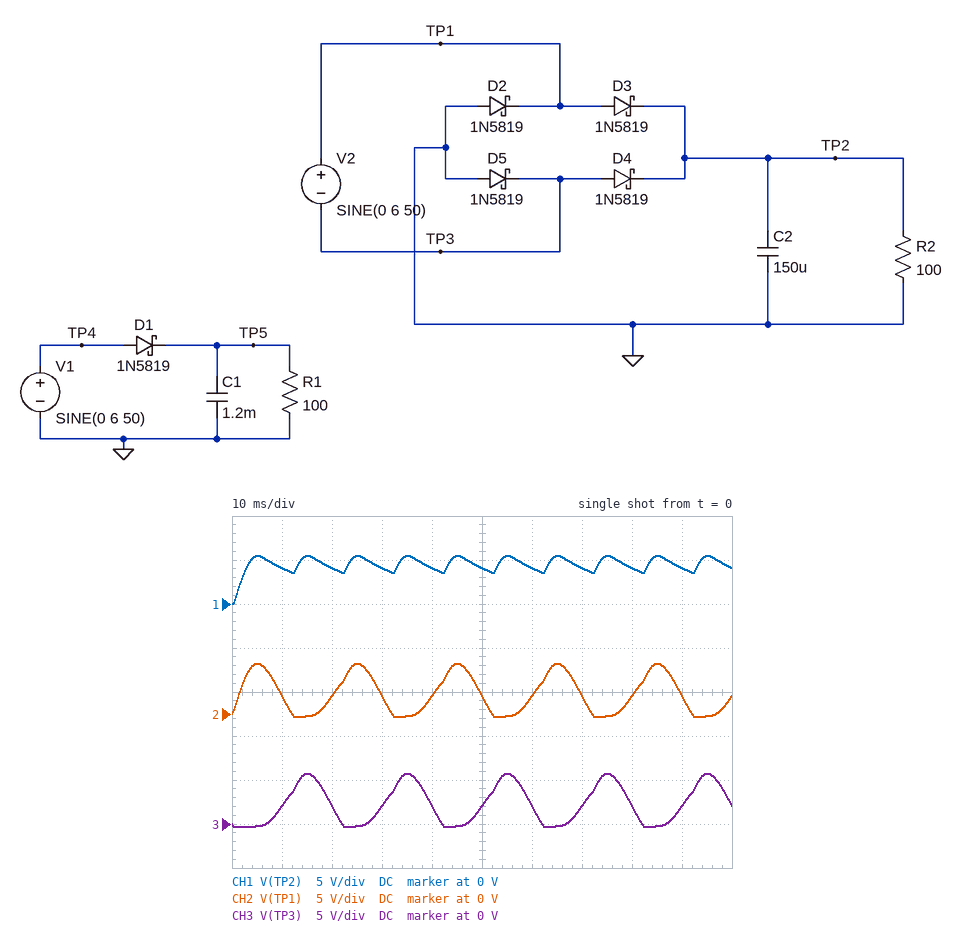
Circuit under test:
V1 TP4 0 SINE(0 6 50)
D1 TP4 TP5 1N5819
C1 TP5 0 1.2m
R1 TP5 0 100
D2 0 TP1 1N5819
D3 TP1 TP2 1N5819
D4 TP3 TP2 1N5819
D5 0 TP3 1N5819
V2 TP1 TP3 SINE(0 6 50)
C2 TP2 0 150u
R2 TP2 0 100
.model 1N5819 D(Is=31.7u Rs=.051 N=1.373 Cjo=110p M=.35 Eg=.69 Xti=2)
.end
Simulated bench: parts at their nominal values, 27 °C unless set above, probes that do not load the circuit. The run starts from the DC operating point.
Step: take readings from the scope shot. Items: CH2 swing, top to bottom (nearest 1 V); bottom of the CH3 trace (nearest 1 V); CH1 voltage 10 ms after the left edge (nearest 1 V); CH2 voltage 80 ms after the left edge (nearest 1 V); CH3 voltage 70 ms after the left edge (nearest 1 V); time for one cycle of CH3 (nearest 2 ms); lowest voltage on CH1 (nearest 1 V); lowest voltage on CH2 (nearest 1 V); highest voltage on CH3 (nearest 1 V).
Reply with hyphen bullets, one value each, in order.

- 6 V
- 0 V
- 4 V
- 2 V
- 2 V
- 20 ms
- 0 V
- 0 V
- 6 V
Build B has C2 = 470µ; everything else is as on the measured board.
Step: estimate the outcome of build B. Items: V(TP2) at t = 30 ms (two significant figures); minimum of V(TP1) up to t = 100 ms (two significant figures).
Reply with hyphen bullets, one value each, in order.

- 4.9 V
- -350 mV
